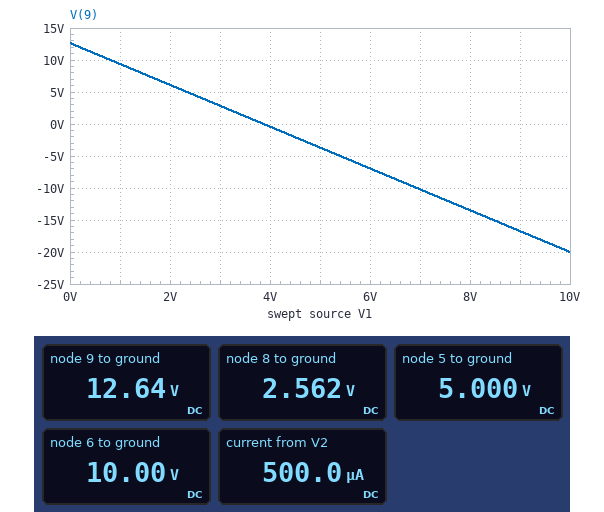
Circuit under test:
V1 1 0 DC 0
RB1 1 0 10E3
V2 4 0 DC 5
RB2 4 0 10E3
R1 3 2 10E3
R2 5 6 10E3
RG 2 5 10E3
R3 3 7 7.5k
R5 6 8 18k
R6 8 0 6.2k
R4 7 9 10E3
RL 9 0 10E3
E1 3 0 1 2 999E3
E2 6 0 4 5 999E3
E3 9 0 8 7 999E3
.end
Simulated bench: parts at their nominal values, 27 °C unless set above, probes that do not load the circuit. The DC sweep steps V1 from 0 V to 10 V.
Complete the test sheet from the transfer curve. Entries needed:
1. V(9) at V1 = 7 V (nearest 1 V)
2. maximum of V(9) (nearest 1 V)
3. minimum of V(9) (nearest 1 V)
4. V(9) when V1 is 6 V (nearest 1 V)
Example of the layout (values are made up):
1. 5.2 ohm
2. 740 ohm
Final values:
1. -10 V
2. 13 V
3. -20 V
4. -7 V
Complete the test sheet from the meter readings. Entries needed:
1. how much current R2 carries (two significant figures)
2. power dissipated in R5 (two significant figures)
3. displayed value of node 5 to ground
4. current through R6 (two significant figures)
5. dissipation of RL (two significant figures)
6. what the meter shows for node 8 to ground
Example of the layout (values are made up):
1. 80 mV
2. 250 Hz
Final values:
1. 500 µA
2. 3.1 mW
3. 5.000 V
4. 410 µA
5. 16 mW
6. 2.562 V
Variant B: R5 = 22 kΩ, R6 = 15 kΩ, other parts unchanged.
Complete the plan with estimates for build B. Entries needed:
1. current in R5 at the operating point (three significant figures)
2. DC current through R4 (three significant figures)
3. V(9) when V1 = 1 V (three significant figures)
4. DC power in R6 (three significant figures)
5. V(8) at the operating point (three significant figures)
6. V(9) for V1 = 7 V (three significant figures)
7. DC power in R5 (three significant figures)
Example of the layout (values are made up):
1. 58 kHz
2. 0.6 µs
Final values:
1. 270 µA
2. 1.21 mA
3. 12.5 V
4. 1.10 mW
5. 4.05 V
6. -9.16 V
7. 1.61 mW
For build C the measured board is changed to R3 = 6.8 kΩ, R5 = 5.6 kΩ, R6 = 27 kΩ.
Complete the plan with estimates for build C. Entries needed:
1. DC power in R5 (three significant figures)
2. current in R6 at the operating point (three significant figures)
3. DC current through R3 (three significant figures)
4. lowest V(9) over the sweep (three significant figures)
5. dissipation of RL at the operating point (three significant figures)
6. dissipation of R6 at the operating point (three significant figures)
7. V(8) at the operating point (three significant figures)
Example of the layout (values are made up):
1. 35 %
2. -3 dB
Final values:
1. 527 µW
2. 307 µA
3. 1.95 mA
4. -22.1 V
5. 77.4 mW
6. 2.54 mW
7. 8.28 V
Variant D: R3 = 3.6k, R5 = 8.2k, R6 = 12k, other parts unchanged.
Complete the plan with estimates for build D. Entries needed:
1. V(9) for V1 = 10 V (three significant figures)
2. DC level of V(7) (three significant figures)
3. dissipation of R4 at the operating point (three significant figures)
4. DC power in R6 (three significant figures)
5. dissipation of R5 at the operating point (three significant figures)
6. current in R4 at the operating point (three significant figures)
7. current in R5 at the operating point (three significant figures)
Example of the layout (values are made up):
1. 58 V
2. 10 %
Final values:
1. -41.7 V
2. 5.94 V
3. 92.4 mW
4. 2.94 mW
5. 2.01 mW
6. 3.04 mA
7. 495 µA
